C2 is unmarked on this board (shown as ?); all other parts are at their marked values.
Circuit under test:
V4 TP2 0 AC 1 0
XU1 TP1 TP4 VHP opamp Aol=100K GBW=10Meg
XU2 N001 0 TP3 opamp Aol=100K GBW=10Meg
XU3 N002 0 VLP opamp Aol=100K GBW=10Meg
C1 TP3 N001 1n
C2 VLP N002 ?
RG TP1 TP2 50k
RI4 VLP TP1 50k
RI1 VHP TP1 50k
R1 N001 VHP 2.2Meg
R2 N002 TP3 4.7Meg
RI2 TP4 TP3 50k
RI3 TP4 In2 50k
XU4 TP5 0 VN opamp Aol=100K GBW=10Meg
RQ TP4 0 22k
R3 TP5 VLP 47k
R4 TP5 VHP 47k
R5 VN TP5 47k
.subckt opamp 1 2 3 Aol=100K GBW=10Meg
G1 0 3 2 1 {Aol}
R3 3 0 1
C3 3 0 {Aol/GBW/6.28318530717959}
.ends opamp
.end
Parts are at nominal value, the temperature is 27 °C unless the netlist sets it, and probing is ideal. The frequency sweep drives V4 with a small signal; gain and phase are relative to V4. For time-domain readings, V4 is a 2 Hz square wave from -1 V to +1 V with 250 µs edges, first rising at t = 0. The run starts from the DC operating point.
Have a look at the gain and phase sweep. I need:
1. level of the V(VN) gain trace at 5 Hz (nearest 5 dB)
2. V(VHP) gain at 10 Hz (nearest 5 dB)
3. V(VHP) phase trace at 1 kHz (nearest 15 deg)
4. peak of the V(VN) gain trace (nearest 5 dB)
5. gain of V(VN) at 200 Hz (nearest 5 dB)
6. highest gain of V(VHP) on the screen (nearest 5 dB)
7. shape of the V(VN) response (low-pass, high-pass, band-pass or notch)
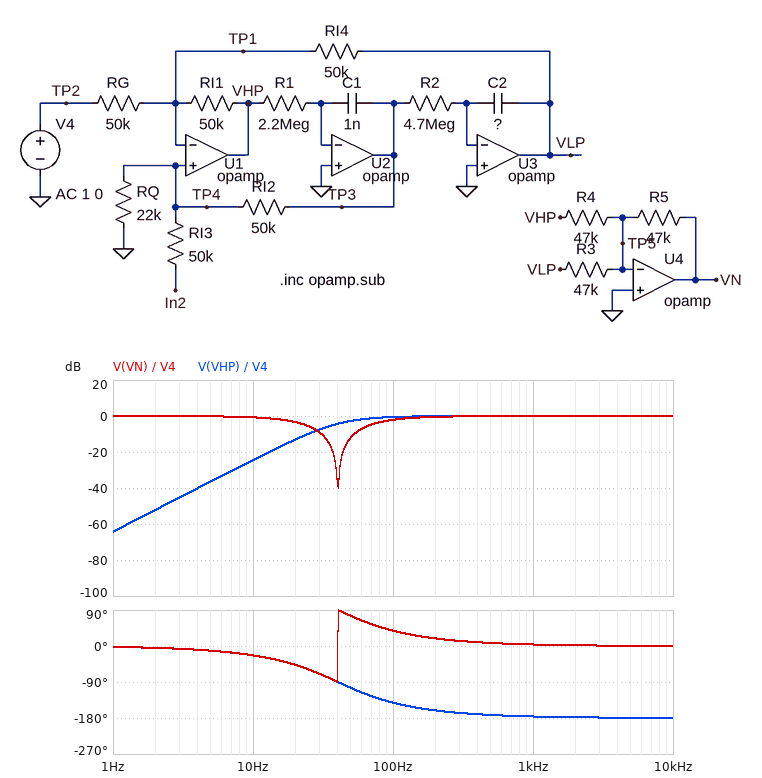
0 dB
-25 dB
-180 deg
0 dB
0 dB
0 dB
notch
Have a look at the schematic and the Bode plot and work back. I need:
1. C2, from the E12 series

1.5 nF
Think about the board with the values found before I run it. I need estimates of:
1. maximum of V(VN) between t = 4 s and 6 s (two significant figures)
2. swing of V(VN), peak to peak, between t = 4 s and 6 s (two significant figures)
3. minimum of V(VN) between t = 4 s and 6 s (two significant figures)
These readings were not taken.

1.0 V
2.0 V
-1.0 V
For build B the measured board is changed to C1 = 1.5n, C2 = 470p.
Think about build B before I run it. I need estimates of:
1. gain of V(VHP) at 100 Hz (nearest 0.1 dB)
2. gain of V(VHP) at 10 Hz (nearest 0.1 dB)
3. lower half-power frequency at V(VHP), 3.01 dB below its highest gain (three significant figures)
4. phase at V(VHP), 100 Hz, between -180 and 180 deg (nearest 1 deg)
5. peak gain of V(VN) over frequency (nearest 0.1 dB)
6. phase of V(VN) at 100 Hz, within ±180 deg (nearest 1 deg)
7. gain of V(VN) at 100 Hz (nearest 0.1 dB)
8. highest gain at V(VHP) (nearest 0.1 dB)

2.1 dB
-30.6 dB
49.6 Hz
-146 deg
0 dB
34 deg
-1.6 dB
3.2 dB
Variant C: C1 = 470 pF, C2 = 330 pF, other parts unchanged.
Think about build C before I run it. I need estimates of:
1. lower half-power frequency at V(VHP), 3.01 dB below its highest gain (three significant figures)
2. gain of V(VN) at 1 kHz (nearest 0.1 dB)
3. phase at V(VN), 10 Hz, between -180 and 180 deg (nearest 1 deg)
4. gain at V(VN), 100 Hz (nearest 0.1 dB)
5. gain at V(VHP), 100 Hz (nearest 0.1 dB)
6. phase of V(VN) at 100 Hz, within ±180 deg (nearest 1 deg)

110 Hz
-0.1 dB
-5 deg
-8.4 dB
-3.7 dB
-68 deg
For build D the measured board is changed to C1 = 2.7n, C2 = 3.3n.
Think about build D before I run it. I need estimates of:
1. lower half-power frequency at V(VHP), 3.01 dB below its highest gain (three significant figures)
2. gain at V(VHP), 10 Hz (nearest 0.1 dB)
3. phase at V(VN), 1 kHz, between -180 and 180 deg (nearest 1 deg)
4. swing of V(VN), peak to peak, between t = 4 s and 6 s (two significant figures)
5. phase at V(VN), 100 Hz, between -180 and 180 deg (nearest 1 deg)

17.4 Hz
-9.6 dB
1 deg
2.1 V
14 deg
